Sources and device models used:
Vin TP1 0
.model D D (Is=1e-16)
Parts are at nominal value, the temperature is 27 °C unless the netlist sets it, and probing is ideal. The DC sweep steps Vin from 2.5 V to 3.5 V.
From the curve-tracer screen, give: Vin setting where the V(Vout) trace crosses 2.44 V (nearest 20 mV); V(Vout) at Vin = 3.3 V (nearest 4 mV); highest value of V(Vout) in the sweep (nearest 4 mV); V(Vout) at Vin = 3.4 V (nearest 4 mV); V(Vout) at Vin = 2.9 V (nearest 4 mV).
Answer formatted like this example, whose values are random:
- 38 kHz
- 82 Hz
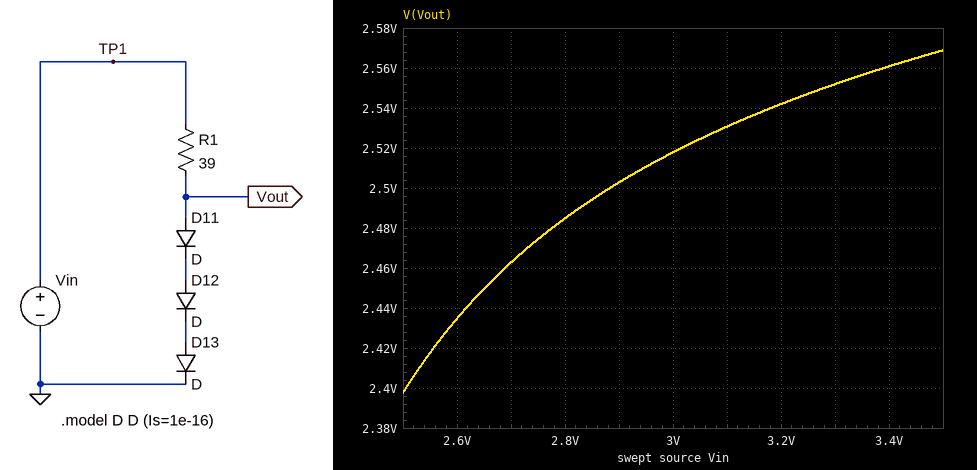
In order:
- 2.62 V
- 2.552 V
- 2.568 V
- 2.560 V
- 2.504 V
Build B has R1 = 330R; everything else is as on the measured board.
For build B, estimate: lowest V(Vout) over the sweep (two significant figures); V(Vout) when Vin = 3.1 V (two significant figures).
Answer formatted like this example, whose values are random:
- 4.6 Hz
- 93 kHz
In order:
- 2.3 V
- 2.4 V
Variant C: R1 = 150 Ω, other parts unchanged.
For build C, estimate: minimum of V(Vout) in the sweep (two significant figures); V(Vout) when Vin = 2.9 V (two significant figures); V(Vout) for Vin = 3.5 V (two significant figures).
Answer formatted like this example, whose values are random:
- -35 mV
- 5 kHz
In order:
- 2.3 V
- 2.4 V
- 2.5 V
